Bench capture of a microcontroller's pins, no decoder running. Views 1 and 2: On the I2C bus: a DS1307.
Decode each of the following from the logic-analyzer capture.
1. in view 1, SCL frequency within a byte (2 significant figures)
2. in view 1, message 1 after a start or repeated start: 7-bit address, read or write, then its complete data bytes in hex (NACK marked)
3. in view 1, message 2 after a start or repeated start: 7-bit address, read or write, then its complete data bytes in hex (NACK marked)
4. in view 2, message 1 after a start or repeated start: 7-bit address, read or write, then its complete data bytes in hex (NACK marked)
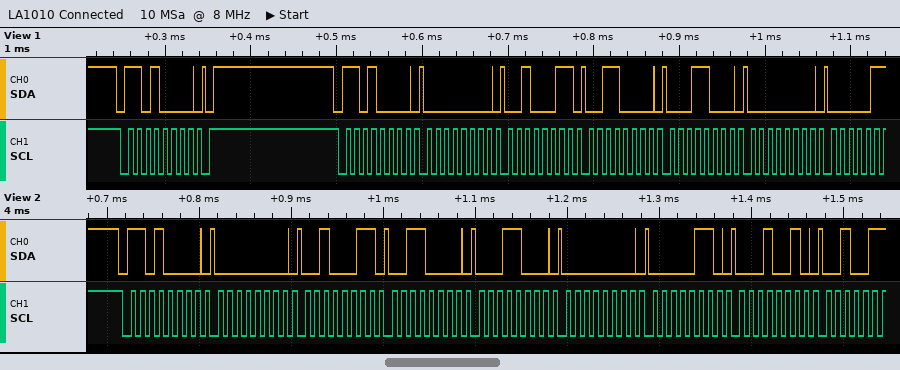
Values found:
100 kHz
0x68 write
0x68 write: 00 23 30 18 00
0x68 write: 00 23 30 18 00 06 12
